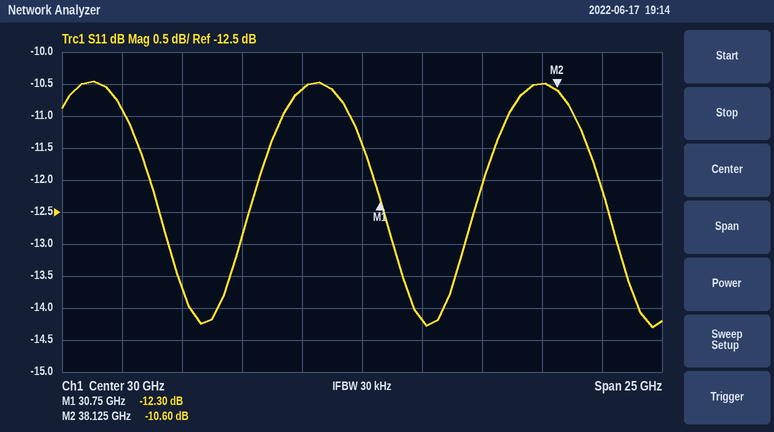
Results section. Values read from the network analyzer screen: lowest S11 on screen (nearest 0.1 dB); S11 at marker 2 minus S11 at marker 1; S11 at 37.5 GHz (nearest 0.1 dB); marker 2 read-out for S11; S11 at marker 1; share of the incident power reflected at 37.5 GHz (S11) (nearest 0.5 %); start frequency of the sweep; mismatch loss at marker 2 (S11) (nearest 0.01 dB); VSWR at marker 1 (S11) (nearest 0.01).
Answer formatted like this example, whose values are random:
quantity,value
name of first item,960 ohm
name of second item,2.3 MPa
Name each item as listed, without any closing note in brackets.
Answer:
quantity,value
lowest S11 on screen,-14.3 dB
S11 at marker 2 minus S11 at marker 1,1.70 dB
S11 at 37.5 GHz,-10.5 dB
marker 2 read-out for S11,-10.60 dB
S11 at marker 1,-12.30 dB
share of the incident power reflected at 37.5 GHz (S11),9.0 %
start frequency of the sweep,17.5 GHz
mismatch loss at marker 2 (S11),0.40 dB
VSWR at marker 1 (S11),1.64
